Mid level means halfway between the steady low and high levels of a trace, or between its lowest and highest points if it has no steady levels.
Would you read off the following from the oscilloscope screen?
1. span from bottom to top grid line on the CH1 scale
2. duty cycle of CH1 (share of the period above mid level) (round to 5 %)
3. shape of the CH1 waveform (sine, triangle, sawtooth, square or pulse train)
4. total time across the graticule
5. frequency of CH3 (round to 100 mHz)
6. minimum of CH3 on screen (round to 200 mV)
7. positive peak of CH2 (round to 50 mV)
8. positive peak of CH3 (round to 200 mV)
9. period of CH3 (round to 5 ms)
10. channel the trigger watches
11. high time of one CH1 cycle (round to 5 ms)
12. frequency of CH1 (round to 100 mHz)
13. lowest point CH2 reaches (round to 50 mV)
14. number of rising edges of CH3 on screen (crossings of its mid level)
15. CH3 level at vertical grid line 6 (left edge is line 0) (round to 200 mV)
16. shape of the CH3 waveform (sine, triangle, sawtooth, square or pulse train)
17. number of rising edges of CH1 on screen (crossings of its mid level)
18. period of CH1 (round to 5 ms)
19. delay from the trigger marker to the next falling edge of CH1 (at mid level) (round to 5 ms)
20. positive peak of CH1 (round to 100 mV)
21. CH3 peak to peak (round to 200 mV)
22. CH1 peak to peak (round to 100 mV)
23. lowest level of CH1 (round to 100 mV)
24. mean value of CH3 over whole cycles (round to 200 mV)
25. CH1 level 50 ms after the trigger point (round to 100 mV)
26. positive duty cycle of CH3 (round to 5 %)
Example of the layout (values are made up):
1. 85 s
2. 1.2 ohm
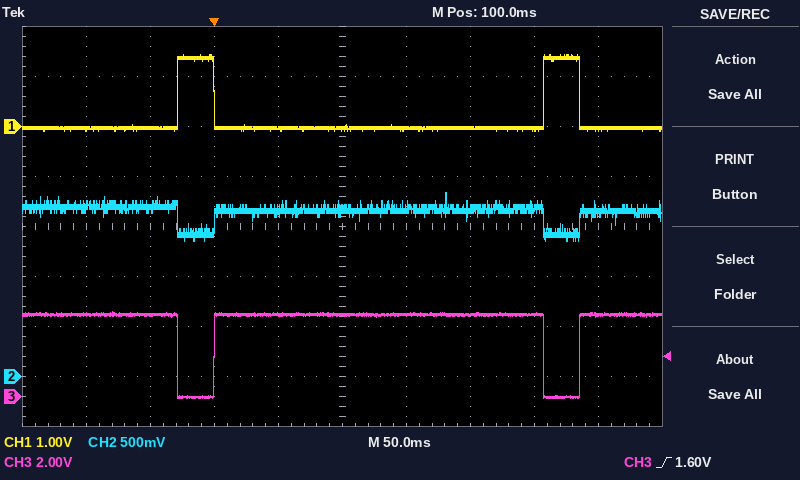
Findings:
1. 8 V
2. 10 %
3. pulse train
4. 500 ms
5. 3.5 Hz
6. 0.0 V
7. 1.85 V
8. 3.4 V
9. 285 ms
10. CH3
11. 30 ms
12. 3.5 Hz
13. 1.35 V
14. 2
15. 3.2 V
16. pulse train
17. 2
18. 285 ms
19. 285 ms
20. 1.4 V
21. 3.4 V
22. 1.5 V
23. -100 mV
24. 3.0 V
25. 0.0 V
26. 90 %
